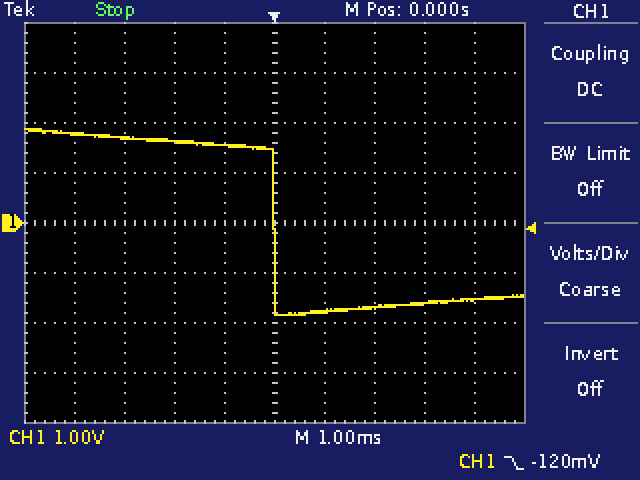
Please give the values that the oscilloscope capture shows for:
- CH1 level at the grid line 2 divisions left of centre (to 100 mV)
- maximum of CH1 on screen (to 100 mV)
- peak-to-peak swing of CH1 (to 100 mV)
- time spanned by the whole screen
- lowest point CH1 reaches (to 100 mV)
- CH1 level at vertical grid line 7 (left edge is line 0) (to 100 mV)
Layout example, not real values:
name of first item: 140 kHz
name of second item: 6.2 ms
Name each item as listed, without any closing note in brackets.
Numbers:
CH1 level at the grid line 2 divisions left of centre: 1.6 V
maximum of CH1 on screen: 1.9 V
peak-to-peak swing of CH1: 3.7 V
time spanned by the whole screen: 10 ms
lowest point CH1 reaches: -1.8 V
CH1 level at vertical grid line 7 (left edge is line 0): -1.7 V
